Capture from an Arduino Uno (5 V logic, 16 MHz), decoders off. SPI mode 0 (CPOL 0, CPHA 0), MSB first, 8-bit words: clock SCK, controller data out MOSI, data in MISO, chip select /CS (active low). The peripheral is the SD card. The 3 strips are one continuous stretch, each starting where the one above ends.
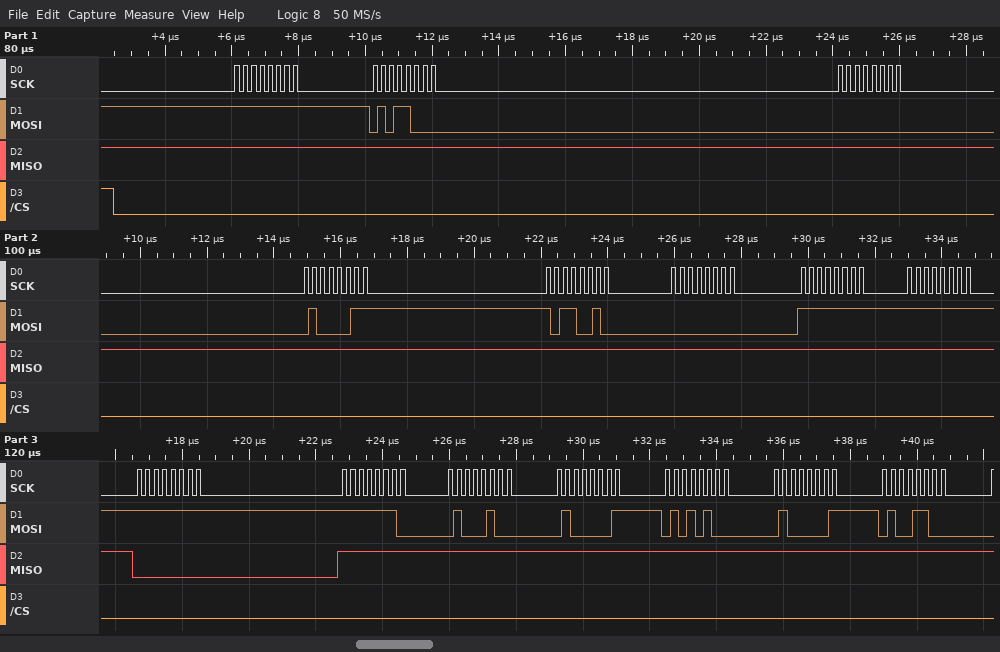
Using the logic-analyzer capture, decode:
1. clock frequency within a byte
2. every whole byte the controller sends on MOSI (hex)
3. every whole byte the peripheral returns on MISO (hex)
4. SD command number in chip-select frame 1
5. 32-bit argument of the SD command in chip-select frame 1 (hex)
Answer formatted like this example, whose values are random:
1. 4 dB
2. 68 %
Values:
1. 4 MHz
2. FF 58 00 43 B2 00 FF FF FF FE 44 41 54 41 4C
3. FF FF FF FF FF FF FF FF 00 FF FF FF FF FF FF
4. CMD24
5. 0x0043B200
